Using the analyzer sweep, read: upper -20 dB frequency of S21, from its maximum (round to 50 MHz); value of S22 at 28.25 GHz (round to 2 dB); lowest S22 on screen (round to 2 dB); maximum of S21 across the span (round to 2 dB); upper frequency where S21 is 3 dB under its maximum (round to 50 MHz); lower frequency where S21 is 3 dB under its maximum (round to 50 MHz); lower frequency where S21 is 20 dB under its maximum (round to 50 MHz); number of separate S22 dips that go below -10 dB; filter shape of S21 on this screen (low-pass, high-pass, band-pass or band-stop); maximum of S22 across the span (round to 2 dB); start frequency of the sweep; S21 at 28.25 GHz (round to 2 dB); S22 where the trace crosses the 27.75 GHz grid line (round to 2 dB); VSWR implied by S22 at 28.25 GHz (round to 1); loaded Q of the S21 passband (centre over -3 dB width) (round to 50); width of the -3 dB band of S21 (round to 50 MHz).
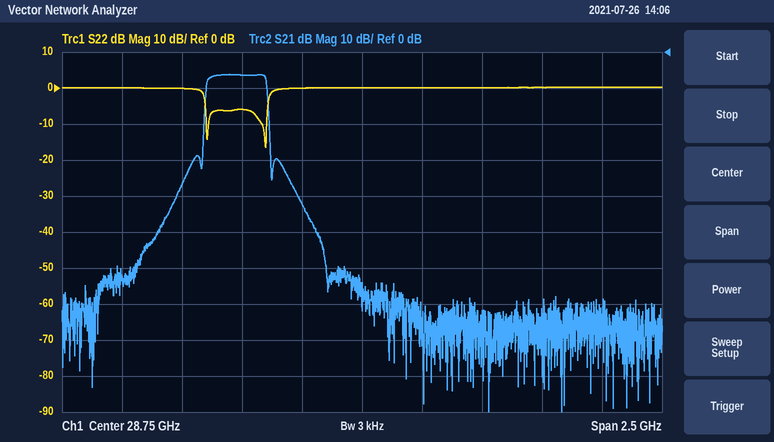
28.35 GHz
-6 dB
-16 dB
-6 dB
28.35 GHz
28.10 GHz
28.10 GHz
2
band-pass
0 dB
27.5 GHz
-6 dB
0 dB
3
100
250 MHz
